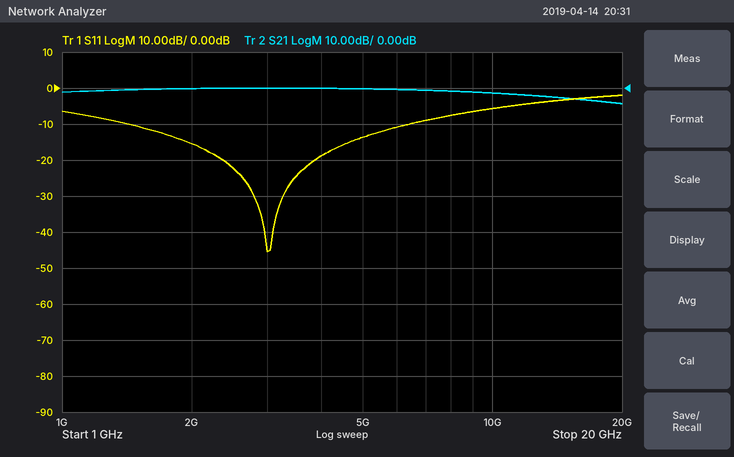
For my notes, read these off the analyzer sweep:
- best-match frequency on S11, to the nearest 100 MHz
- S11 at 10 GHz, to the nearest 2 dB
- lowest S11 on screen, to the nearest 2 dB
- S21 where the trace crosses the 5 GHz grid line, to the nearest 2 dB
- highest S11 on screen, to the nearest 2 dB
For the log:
3.0 GHz
-6 dB
-46 dB
0 dB
-2 dB
